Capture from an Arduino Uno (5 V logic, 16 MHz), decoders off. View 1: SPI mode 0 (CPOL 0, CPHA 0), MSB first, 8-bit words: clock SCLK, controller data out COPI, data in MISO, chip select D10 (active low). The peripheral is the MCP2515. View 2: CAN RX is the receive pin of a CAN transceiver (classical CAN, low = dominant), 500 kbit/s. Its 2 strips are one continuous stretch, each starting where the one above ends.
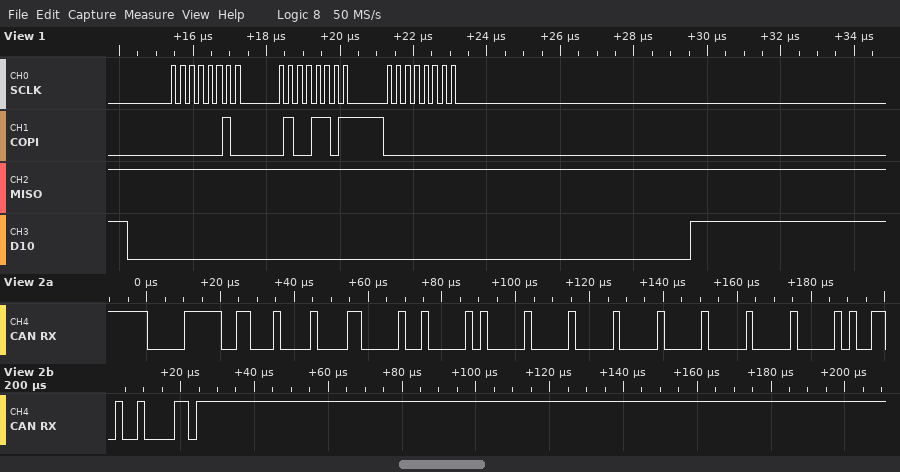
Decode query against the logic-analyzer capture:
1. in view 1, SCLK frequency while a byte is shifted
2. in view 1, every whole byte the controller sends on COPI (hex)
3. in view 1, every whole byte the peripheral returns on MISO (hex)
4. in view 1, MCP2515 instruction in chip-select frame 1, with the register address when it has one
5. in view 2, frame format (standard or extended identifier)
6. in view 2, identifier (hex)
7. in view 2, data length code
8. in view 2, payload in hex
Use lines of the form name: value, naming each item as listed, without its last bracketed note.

in view 1, SCLK frequency while a byte is shifted: 4 MHz
in view 1, every whole byte the controller sends on COPI: 0x02 0x4D 0x00
in view 1, every whole byte the peripheral returns on MISO: 0xFF 0xFF 0xFF
in view 1, MCP2515 instruction in chip-select frame 1, with the register address when it has one: WRITE 0x4D
in view 2, frame format: standard
in view 2, identifier: 0x07B
in view 2, data length code: 8
in view 2, payload in hex: 43 01 02 00 00 00 00 00
